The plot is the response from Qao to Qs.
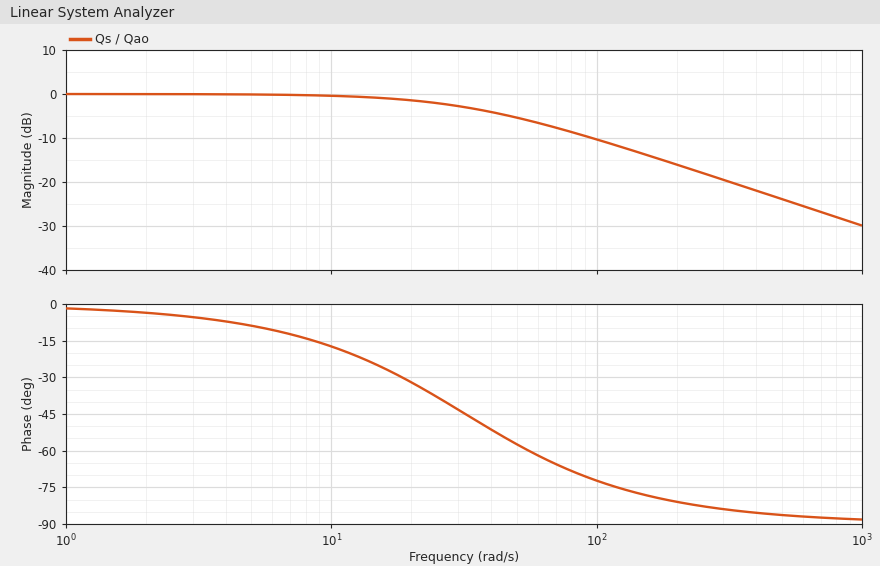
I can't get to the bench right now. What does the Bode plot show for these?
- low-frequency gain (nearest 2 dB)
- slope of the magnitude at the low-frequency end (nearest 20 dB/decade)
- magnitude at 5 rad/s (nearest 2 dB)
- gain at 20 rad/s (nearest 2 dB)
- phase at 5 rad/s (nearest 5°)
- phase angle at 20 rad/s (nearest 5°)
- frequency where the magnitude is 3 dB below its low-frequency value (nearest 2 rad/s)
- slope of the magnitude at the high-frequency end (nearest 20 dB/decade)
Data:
0 dB
0 dB/decade
0 dB
-2 dB
-10°
-30°
32 rad/s
-20 dB/decade
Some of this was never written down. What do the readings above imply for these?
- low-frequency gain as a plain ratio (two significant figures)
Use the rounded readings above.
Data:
1.0
